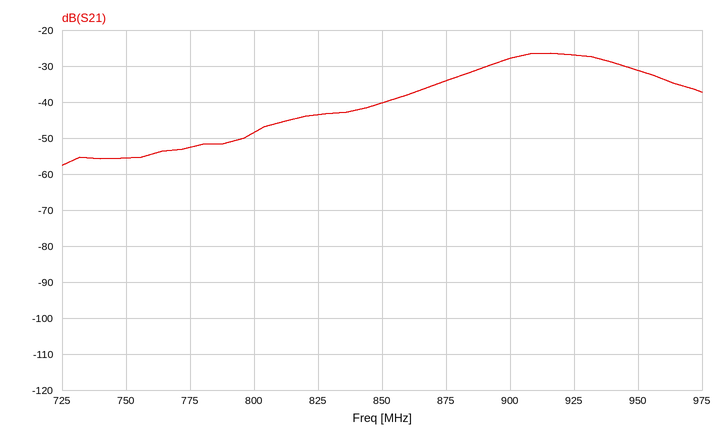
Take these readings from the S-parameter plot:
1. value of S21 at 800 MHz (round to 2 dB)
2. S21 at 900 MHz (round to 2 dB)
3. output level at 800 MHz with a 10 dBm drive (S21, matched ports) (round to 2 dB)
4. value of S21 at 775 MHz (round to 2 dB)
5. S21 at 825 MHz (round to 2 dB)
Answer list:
-48 dB
-28 dB
-38 dBm
-52 dB
-44 dB
